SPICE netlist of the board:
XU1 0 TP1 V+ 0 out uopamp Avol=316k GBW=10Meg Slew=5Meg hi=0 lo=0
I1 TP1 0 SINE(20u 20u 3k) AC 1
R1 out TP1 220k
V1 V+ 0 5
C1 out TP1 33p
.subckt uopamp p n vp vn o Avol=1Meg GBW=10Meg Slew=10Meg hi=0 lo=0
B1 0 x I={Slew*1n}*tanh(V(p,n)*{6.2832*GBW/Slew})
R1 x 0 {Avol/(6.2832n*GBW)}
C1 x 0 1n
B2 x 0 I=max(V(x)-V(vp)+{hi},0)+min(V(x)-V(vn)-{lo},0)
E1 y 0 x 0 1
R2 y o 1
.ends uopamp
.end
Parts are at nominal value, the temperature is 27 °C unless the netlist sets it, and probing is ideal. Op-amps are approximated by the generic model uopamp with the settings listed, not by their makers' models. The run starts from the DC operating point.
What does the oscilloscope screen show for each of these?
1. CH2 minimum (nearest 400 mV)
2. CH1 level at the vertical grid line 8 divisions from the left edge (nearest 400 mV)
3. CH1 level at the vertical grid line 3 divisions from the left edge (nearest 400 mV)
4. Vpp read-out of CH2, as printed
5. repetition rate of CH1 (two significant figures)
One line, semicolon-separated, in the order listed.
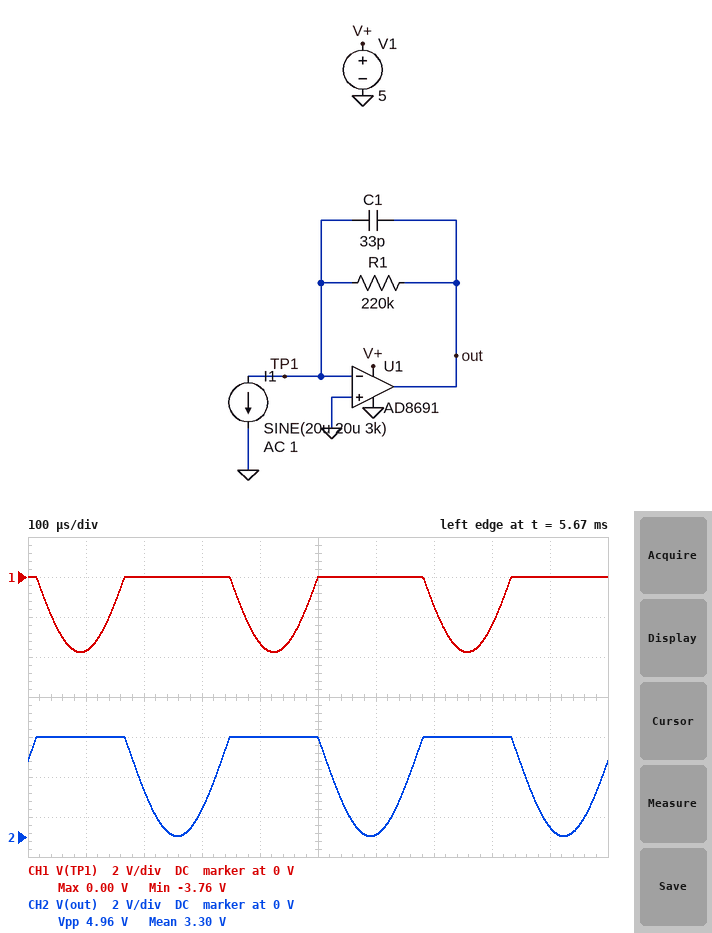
0 V; -2.4 V; 0 V; 4.96 V; 3.0 kHz
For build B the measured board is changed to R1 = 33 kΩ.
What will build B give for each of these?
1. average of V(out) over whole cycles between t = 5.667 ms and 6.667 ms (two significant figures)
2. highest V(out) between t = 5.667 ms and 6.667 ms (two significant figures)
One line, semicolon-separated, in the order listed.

660 mV; 1.3 V
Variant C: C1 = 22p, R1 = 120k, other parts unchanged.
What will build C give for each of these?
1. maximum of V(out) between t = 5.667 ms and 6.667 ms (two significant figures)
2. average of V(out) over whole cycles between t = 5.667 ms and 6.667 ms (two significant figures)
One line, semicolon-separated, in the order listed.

4.8 V; 2.4 V
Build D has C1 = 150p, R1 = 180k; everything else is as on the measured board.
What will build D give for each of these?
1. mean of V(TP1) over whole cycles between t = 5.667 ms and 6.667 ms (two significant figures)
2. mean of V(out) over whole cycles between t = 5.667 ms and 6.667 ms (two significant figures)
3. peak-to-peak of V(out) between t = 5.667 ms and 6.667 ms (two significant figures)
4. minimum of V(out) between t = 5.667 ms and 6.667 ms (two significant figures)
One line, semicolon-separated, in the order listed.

-420 mV; 3.2 V; 4.6 V; 390 mV
